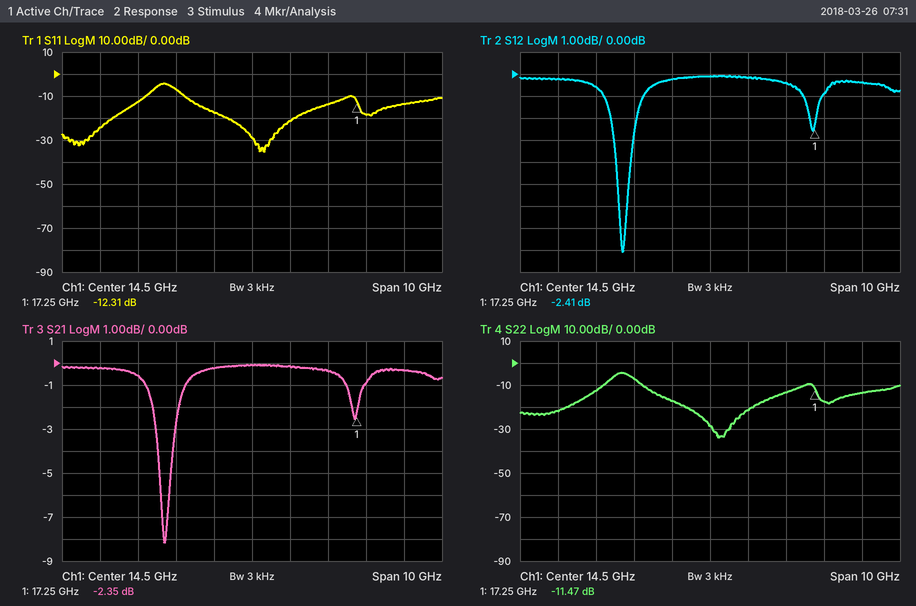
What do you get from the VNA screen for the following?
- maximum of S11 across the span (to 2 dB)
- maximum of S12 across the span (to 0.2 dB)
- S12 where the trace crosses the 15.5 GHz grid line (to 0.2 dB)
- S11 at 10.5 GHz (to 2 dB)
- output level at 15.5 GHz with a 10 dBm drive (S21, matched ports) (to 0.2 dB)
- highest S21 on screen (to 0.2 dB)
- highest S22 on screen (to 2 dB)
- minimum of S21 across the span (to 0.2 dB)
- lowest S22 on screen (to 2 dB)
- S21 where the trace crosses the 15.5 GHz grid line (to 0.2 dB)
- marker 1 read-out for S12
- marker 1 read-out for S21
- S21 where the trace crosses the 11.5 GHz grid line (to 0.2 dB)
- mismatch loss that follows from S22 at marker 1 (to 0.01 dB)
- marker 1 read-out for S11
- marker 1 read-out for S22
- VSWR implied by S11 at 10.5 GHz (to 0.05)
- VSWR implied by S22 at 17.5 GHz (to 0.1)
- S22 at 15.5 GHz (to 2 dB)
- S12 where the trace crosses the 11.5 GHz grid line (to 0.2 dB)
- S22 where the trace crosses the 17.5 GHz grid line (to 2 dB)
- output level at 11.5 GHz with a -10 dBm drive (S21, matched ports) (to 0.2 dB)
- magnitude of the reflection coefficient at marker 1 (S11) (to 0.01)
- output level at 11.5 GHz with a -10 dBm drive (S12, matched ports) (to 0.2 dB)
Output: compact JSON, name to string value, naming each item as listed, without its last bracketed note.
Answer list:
{"maximum of S11 across the span": "-4 dB", "maximum of S12 across the span": "0.0 dB", "S12 where the trace crosses the 15.5 GHz grid line": "-0.2 dB", "S11 at 10.5 GHz": "-24 dB", "output level at 15.5 GHz with a 10 dBm drive (S21, matched ports)": "9.8 dBm", "highest S21 on screen": "0.0 dB", "highest S22 on screen": "-4 dB", "minimum of S21 across the span": "-8.2 dB", "lowest S22 on screen": "-34 dB", "S21 where the trace crosses the 15.5 GHz grid line": "-0.2 dB", "marker 1 read-out for S12": "-2.41 dB", "marker 1 read-out for S21": "-2.35 dB", "S21 where the trace crosses the 11.5 GHz grid line": "-0.6 dB", "mismatch loss that follows from S22 at marker 1": "0.32 dB", "marker 1 read-out for S11": "-12.31 dB", "marker 1 read-out for S22": "-11.47 dB", "VSWR implied by S11 at 10.5 GHz": "1.15", "VSWR implied by S22 at 17.5 GHz": "1.3", "S22 at 15.5 GHz": "-22 dB", "S12 where the trace crosses the 11.5 GHz grid line": "-0.6 dB", "S22 where the trace crosses the 17.5 GHz grid line": "-18 dB", "output level at 11.5 GHz with a -10 dBm drive (S21, matched ports)": "-10.6 dBm", "magnitude of the reflection coefficient at marker 1 (S11)": "0.24", "output level at 11.5 GHz with a -10 dBm drive (S12, matched ports)": "-10.6 dBm"}
